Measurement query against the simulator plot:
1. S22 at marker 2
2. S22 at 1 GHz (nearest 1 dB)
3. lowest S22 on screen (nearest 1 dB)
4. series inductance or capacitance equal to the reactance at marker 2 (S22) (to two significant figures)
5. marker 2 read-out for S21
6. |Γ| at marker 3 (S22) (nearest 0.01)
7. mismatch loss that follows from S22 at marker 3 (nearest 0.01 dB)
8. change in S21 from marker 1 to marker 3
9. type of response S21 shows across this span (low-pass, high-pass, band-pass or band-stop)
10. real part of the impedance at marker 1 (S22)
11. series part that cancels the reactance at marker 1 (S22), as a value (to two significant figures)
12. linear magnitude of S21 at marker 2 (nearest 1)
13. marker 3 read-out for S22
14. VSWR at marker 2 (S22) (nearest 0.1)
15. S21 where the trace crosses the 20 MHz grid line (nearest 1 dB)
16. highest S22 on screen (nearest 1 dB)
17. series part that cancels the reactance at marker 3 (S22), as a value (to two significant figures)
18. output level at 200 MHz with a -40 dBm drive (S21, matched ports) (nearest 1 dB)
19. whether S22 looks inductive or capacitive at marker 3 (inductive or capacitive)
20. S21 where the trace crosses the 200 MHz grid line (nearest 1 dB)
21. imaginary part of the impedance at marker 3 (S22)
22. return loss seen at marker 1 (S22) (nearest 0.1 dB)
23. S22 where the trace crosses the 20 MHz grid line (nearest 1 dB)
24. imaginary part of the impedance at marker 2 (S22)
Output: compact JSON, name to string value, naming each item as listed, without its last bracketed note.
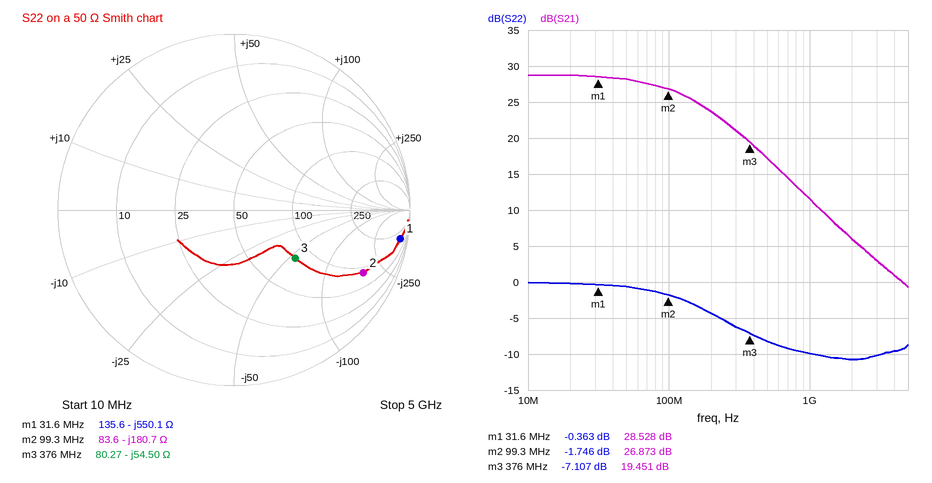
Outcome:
{"S22 at marker 2": "-1.746 dB", "S22 at 1 GHz": "-10 dB", "lowest S22 on screen": "-11 dB", "series inductance or capacitance equal to the reactance at marker 2 (S22)": "8.9 pF", "marker 2 read-out for S21": "26.873 dB", "|Γ| at marker 3 (S22)": "0.44", "mismatch loss that follows from S22 at marker 3": "0.94 dB", "change in S21 from marker 1 to marker 3": "-9.077 dB", "type of response S21 shows across this span": "low-pass", "real part of the impedance at marker 1": "135.6 Ω", "series part that cancels the reactance at marker 1 (S22), as a value": "2.8 µH", "linear magnitude of S21 at marker 2": "22", "marker 3 read-out for S22": "-7.107 dB", "VSWR at marker 2 (S22)": "10.0", "S21 where the trace crosses the 20 MHz grid line": "29 dB", "highest S22 on screen": "0 dB", "series part that cancels the reactance at marker 3 (S22), as a value": "23 nH", "output level at 200 MHz with a -40 dBm drive (S21, matched ports)": "-16 dBm", "whether S22 looks inductive or capacitive at marker 3": "capacitive", "S21 where the trace crosses the 200 MHz grid line": "24 dB", "imaginary part of the impedance at marker 3": "-54.50 Ω", "return loss seen at marker 1 (S22)": "0.4 dB", "S22 where the trace crosses the 20 MHz grid line": "0 dB", "imaginary part of the impedance at marker 2": "-180.7 Ω"}
